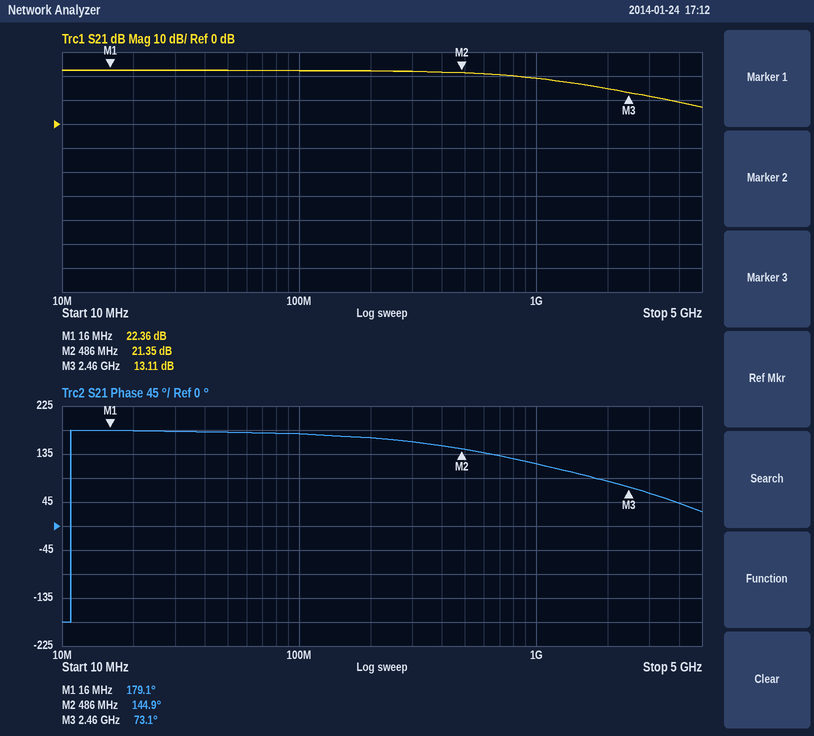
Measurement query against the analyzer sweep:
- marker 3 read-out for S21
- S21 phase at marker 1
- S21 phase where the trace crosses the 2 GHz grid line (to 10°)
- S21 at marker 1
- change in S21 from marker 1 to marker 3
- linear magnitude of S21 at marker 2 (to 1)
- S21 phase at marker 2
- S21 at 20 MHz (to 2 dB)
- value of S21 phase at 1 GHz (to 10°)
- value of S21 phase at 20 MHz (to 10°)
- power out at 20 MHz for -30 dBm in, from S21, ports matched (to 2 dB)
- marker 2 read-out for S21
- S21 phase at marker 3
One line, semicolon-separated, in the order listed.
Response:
13.11 dB; 179.1°; 80°; 22.36 dB; -9.25 dB; 12; 144.9°; 22 dB; 120°; 180°; -8 dBm; 21.35 dB; 73.1°
